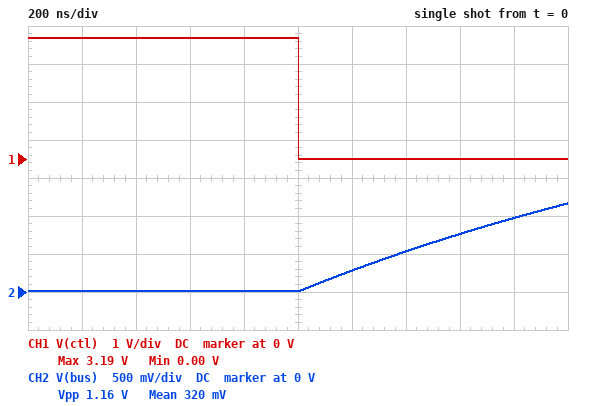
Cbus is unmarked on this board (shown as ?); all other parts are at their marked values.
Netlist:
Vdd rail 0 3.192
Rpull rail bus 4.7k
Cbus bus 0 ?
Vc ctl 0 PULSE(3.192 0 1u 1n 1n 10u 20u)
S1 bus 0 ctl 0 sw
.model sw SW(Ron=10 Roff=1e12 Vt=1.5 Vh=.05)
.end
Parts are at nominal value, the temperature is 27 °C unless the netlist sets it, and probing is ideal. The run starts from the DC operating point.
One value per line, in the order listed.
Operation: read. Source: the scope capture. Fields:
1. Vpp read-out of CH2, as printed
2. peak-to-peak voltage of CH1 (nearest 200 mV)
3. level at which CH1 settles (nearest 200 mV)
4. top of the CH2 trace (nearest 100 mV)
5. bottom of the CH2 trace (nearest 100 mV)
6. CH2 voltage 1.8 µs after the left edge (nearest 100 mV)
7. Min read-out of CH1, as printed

1.16 V
3.2 V
0 V
1.2 V
0 V
1.0 V
0.00 V
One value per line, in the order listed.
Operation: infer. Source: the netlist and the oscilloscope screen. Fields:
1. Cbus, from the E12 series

470 pF
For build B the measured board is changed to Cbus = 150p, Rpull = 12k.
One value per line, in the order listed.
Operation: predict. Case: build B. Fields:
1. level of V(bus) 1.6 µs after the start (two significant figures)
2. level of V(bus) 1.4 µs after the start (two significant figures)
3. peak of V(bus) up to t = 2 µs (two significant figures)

910 mV
640 mV
1.4 V
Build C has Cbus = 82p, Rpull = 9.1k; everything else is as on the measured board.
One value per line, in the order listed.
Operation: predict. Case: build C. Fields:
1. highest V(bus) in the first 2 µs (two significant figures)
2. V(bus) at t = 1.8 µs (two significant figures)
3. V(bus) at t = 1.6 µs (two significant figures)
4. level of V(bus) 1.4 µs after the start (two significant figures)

2.4 V
2.1 V
1.8 V
1.3 V
